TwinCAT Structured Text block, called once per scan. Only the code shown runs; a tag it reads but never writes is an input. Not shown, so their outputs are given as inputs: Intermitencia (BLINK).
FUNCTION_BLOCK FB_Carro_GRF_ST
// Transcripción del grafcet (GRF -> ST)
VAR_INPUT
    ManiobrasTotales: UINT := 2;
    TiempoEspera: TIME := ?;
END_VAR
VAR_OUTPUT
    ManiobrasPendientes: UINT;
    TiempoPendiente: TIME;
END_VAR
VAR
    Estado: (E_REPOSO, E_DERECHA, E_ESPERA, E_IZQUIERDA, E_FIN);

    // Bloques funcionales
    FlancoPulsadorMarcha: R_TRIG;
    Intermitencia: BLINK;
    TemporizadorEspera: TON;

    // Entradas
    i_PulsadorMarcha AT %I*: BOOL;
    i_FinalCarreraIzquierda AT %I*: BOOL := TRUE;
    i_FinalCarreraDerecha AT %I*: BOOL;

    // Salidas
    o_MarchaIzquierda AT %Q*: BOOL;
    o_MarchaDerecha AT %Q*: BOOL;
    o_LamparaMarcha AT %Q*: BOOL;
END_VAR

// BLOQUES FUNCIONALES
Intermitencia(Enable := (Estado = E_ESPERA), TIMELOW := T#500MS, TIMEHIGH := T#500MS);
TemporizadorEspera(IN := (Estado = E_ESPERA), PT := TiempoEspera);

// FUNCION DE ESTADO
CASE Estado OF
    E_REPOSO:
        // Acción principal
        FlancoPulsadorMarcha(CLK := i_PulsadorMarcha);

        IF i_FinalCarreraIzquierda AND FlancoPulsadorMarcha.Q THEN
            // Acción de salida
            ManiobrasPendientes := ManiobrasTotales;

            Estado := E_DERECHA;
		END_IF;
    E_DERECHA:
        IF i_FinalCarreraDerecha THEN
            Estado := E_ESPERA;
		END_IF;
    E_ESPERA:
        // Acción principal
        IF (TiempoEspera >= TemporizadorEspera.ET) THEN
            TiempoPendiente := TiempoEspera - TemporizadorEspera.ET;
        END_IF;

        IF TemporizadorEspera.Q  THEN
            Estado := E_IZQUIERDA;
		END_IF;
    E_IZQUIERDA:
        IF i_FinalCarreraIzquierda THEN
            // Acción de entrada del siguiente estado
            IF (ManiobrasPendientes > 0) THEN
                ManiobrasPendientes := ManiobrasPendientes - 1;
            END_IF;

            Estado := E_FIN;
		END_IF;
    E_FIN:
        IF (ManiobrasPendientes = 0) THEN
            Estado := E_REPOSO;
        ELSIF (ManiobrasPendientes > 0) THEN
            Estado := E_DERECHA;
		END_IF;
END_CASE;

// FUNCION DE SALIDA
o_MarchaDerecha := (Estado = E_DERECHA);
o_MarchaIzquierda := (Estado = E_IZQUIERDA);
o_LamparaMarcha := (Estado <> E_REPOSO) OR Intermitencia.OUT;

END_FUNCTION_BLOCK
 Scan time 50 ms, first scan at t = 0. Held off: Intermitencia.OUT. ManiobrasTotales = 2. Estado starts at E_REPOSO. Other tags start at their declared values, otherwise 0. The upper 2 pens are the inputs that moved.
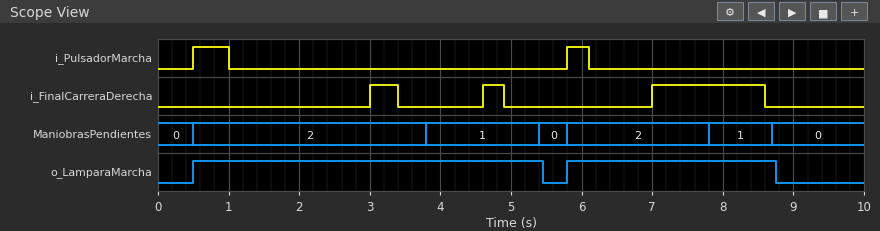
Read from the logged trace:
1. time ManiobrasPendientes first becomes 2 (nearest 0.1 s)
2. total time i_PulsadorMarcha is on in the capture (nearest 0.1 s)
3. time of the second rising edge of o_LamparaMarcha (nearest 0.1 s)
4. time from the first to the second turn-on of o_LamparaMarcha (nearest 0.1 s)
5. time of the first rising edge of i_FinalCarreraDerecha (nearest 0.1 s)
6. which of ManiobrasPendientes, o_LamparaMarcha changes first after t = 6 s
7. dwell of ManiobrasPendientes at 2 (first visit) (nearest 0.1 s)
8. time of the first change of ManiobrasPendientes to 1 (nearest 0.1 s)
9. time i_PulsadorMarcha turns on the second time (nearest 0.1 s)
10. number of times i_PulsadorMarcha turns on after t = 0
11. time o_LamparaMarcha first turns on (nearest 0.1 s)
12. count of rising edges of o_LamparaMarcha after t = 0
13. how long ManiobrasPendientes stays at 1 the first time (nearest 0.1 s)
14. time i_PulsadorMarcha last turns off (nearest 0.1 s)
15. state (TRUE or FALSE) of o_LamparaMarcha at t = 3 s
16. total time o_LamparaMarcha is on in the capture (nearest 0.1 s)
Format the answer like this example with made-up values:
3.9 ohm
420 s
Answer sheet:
0.5 s
0.8 s
5.8 s
5.3 s
3.0 s
ManiobrasPendientes
3.3 s
3.8 s
5.8 s
2
0.5 s
2
1.6 s
6.1 s
TRUE
7.9 s
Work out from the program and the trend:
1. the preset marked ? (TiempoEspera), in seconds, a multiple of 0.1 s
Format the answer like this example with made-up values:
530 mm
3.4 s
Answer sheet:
0.7 s
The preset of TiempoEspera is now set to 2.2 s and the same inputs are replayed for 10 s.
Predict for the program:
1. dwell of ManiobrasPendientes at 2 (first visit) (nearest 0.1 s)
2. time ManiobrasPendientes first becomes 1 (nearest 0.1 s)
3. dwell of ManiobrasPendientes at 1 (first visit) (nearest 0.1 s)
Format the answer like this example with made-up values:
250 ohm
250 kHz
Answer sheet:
4.8 s
5.3 s
4.0 s
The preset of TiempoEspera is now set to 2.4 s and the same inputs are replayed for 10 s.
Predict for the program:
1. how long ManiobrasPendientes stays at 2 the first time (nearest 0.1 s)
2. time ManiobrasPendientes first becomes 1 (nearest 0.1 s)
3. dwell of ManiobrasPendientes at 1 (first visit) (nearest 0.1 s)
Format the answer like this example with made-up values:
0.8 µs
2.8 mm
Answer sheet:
5.0 s
5.5 s
4.0 s
